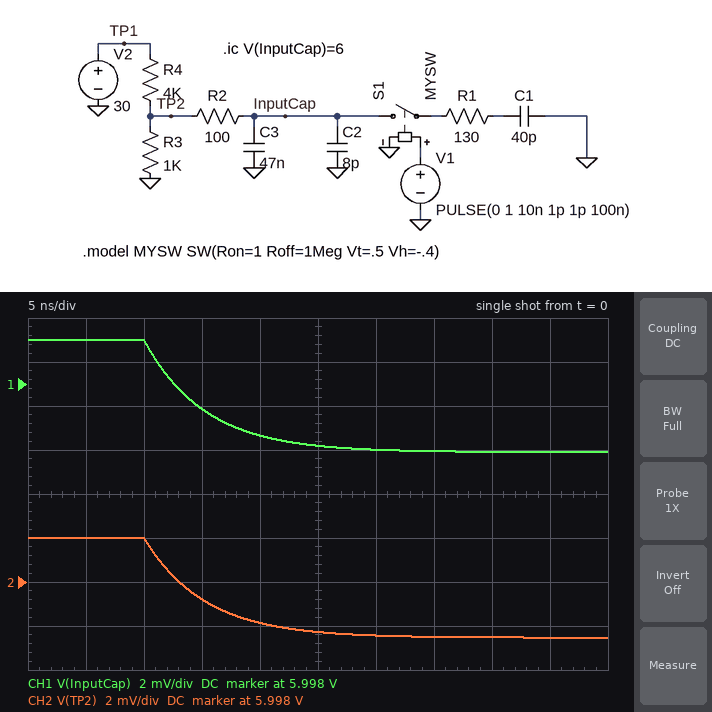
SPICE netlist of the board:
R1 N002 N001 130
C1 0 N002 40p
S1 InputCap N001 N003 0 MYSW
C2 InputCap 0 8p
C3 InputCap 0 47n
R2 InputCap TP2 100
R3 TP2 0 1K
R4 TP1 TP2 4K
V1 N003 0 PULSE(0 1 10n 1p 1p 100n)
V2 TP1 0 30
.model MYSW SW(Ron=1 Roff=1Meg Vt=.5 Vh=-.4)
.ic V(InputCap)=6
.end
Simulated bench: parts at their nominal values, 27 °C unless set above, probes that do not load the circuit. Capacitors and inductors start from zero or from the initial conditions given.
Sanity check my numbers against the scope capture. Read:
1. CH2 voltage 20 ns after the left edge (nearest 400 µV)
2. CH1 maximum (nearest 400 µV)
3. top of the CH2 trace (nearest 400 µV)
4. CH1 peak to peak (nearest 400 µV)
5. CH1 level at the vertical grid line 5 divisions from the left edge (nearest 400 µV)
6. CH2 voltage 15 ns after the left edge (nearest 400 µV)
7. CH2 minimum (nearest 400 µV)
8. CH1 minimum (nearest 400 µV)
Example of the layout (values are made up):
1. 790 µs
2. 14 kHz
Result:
1. 5.9960 V
2. 6.0000 V
3. 6.0000 V
4. 5.2 mV
5. 5.9952 V
6. 5.9972 V
7. 5.9956 V
8. 5.9948 V
